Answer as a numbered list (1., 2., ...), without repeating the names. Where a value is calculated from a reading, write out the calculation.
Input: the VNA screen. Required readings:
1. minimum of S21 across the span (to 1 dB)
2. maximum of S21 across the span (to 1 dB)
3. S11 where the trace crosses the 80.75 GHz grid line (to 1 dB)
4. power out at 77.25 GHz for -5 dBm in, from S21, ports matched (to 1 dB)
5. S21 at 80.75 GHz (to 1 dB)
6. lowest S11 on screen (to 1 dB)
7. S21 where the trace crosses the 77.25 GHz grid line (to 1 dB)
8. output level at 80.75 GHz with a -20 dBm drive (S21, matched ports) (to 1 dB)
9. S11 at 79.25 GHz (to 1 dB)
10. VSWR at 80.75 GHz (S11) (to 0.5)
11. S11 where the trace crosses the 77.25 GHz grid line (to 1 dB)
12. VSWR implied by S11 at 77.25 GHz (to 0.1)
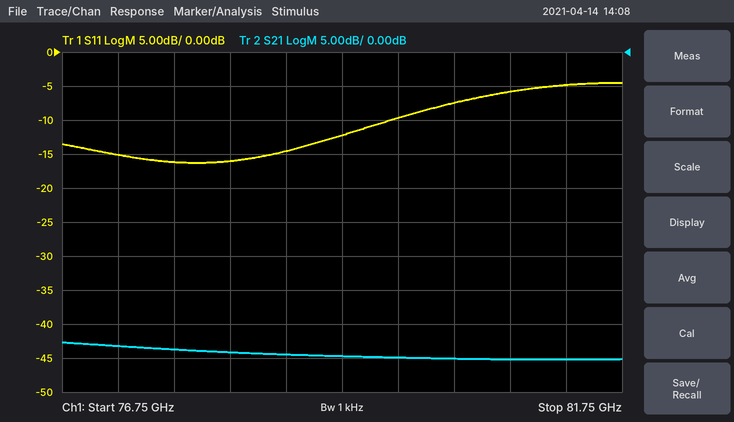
1. -45 dB
2. -43 dB
3. -6 dB
4. -5 dBm + (-43 dB) = -48 dBm
5. -45 dB
6. -16 dB
7. -43 dB
8. -20 dBm + (-45 dB) = -65 dBm
9. -12 dB
10. |Γ| = 10^(-6/20) = 0.5012; VSWR = (1 + 0.5012)/(1 − 0.5012) ≈ 3.0
11. -15 dB
12. |Γ| = 10^(-15/20) = 0.1778; VSWR = (1 + 0.1778)/(1 − 0.1778) ≈ 1.4
